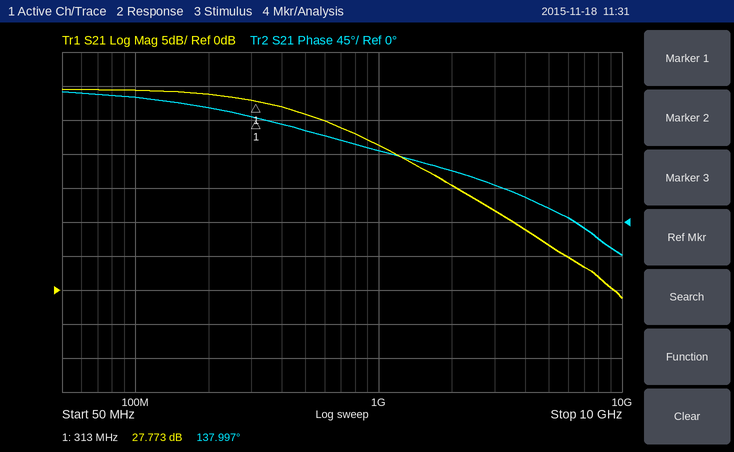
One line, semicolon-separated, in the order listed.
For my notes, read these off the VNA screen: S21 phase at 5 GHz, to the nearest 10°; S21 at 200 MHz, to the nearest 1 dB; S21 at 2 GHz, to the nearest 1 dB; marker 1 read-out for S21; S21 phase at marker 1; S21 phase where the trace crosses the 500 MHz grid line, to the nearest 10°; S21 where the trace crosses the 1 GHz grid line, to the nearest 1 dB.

20°; 29 dB; 15 dB; 27.773 dB; 137.997°; 120°; 21 dB
